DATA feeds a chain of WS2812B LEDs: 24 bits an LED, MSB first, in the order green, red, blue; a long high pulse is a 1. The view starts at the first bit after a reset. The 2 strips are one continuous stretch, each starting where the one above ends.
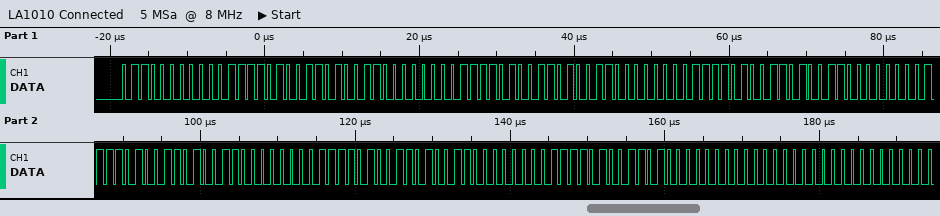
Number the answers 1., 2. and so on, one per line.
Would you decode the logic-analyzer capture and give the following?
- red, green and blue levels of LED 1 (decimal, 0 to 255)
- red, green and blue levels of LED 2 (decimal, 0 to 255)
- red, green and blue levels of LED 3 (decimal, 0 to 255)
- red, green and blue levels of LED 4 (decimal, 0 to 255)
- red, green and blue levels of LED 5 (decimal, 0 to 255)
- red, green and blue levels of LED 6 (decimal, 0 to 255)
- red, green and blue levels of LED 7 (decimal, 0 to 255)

1. 30, 96, 154
2. 30, 96, 154
3. 30, 96, 154
4. 30, 96, 154
5. 30, 96, 154
6. 30, 96, 154
7. 0, 0, 0
